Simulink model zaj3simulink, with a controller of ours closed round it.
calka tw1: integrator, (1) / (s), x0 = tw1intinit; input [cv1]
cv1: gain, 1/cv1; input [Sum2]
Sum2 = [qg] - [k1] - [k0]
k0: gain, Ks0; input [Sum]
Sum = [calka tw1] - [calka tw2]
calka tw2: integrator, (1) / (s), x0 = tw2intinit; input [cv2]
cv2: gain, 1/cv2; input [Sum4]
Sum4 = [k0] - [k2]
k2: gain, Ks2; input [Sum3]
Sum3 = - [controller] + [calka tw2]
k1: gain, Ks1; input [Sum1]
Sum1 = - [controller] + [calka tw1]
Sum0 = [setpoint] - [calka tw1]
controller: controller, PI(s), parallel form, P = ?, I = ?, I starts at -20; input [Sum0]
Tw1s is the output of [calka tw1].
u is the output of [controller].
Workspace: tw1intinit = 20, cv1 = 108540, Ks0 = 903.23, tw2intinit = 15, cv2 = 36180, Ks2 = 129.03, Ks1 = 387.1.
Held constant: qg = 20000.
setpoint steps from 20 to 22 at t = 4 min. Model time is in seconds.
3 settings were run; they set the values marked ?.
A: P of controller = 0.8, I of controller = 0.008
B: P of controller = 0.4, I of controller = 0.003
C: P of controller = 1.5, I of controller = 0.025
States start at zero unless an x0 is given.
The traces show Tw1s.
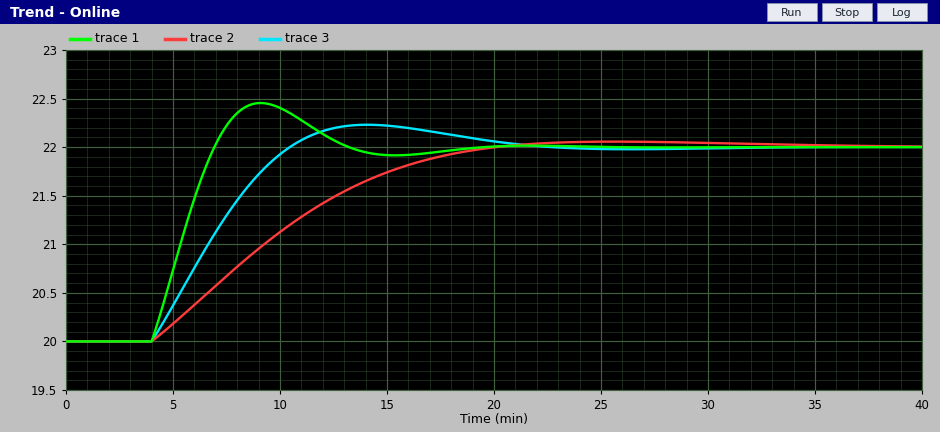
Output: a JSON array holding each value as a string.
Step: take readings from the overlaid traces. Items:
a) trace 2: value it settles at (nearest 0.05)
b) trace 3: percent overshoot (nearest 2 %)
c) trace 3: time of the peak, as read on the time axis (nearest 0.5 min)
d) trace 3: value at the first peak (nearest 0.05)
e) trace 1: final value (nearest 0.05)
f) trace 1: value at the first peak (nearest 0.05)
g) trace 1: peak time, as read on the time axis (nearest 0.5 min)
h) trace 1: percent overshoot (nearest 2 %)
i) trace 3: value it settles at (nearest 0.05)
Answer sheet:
["22.00", "12 %", "14.0 min", "22.25", "22.00", "22.45", "9.0 min", "22 %", "22.00"]
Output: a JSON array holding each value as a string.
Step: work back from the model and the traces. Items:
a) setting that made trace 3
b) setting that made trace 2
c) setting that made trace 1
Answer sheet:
["A", "B", "C"]
